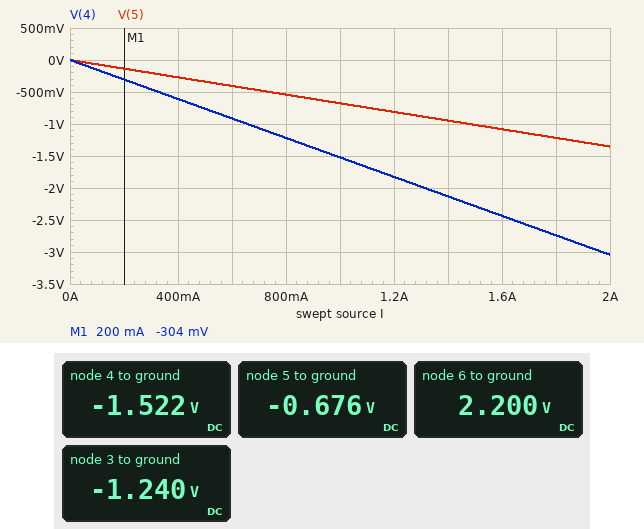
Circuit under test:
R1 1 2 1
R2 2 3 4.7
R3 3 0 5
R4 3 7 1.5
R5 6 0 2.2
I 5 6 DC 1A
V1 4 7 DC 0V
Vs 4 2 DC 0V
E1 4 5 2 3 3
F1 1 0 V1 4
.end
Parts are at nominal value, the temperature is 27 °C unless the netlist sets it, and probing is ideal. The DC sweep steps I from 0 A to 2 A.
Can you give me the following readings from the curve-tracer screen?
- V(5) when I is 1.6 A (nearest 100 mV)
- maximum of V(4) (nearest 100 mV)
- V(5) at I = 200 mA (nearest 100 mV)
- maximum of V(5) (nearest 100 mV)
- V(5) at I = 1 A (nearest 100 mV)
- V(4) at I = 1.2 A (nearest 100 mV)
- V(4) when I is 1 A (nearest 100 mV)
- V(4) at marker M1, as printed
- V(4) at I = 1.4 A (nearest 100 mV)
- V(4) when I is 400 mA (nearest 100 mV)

-1.1 V
0 V
-100 mV
0 V
-700 mV
-1.8 V
-1.5 V
-304 mV
-2.1 V
-600 mV
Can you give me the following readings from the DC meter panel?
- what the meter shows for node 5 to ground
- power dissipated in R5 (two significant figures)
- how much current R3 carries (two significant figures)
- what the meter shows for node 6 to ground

-0.676 V
2.2 W
250 mA
2.200 V
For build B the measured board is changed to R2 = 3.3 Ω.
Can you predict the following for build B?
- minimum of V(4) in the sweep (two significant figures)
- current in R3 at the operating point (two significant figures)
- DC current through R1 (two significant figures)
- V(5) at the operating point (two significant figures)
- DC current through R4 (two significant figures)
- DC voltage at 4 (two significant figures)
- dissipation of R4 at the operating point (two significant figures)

-3.2 V
270 mA
730 mA
-780 mV
180 mA
-1.6 V
50 mW
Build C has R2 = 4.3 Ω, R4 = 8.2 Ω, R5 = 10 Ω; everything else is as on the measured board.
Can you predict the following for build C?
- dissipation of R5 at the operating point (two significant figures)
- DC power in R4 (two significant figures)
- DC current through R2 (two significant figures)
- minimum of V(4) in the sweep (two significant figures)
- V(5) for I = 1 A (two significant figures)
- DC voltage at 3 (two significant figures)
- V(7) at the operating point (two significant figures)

10 W
170 mW
280 mA
-6.6 V
270 mV
-2.1 V
-3.3 V
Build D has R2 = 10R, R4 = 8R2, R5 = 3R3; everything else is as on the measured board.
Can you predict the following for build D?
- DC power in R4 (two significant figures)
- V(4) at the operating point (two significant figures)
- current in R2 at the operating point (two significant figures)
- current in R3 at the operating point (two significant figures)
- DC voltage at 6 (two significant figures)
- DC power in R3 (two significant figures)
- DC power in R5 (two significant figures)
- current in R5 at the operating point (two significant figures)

240 mW
-3.0 V
140 mA
310 mA
3.3 V
490 mW
3.3 W
1.0 A
